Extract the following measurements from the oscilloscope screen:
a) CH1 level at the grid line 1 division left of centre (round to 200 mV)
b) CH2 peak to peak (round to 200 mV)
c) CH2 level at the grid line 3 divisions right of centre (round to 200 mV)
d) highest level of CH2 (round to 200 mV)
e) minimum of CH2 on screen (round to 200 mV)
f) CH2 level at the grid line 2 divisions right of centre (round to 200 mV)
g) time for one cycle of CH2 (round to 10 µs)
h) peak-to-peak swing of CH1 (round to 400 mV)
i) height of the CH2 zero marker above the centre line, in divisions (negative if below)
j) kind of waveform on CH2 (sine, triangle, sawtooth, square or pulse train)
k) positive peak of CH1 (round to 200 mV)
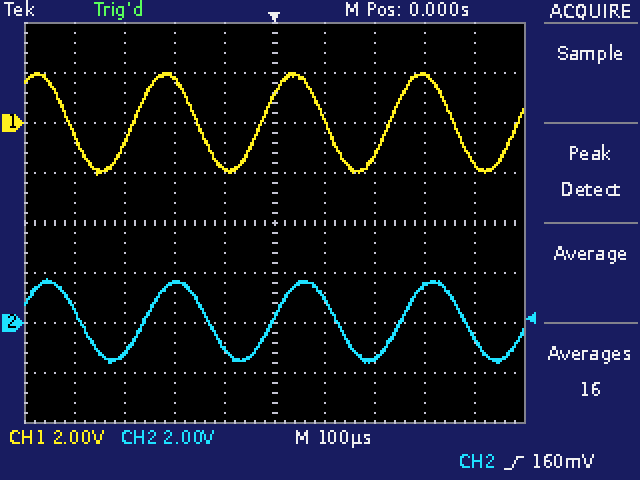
-1.8 V
3.4 V
1.4 V
1.8 V
-1.6 V
-1.4 V
260 µs
4.0 V
-2.0 div
sine
2.0 V
